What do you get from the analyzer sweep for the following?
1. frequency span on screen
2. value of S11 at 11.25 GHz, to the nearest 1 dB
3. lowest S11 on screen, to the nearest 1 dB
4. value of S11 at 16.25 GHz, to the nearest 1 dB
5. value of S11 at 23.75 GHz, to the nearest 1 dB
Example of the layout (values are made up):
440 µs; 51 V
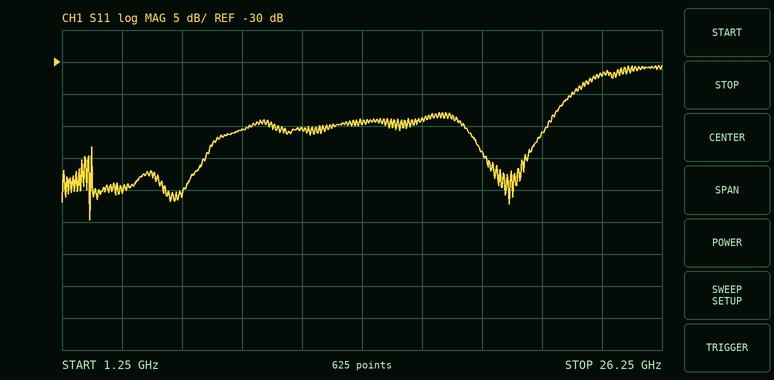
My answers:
25 GHz; -40 dB; -55 dB; -39 dB; -32 dB
